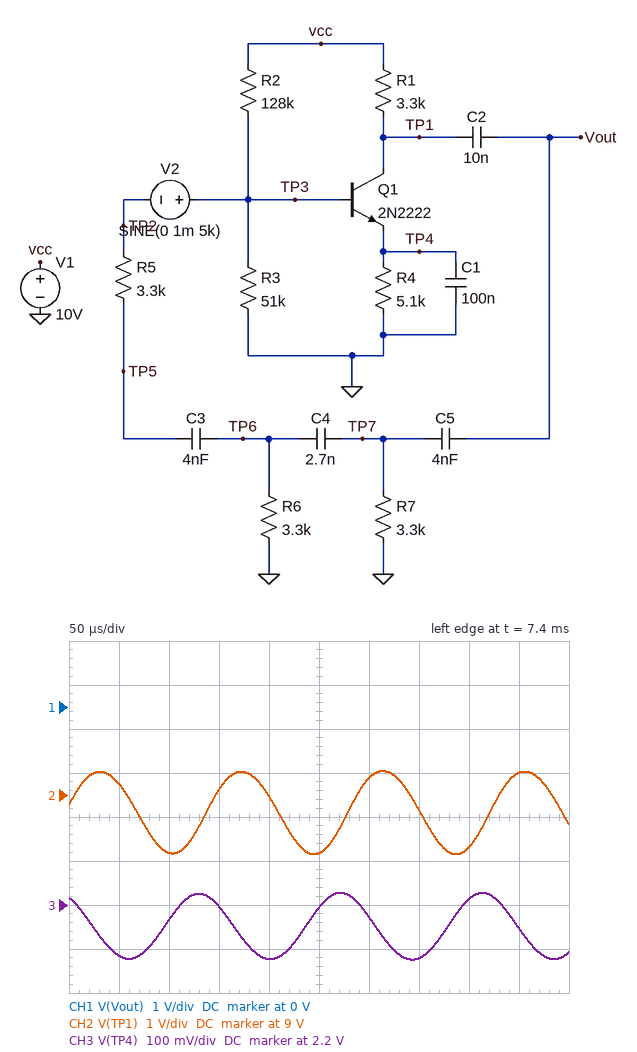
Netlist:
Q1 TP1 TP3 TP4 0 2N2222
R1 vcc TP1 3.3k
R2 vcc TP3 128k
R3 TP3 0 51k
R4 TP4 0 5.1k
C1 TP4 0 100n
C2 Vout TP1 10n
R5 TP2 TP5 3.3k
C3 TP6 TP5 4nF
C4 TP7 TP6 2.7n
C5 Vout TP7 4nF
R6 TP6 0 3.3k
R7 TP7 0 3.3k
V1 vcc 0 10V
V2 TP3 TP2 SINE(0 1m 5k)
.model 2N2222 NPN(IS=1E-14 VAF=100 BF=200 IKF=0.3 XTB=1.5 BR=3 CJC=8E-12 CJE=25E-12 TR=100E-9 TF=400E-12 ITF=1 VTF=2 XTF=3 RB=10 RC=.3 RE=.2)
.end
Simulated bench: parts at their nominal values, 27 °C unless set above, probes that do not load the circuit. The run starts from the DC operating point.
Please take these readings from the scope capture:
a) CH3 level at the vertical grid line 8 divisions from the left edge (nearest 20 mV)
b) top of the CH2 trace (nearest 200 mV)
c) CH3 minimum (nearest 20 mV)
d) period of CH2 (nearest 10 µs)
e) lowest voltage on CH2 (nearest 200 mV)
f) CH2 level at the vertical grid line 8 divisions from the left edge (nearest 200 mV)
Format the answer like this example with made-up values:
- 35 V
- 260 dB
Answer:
- 2.22 V
- 9.6 V
- 2.08 V
- 140 µs
- 7.6 V
- 7.8 V
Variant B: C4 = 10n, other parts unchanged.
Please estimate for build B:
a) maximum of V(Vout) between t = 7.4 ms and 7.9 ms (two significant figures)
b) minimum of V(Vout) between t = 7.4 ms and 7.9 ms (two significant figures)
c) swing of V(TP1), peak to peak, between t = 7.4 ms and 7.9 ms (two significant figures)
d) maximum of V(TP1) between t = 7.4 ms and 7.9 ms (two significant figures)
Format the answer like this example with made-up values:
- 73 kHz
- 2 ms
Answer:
- 6.2 V
- 6.1 V
- 100 mV
- 8.7 V
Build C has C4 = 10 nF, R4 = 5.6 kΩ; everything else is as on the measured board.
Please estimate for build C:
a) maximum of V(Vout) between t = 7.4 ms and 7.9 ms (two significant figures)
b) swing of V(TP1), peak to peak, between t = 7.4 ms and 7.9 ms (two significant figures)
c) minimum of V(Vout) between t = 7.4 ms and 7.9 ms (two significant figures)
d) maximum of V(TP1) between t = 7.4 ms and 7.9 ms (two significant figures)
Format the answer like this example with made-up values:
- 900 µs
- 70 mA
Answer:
- 6.3 V
- 96 mV
- 6.2 V
- 8.8 V
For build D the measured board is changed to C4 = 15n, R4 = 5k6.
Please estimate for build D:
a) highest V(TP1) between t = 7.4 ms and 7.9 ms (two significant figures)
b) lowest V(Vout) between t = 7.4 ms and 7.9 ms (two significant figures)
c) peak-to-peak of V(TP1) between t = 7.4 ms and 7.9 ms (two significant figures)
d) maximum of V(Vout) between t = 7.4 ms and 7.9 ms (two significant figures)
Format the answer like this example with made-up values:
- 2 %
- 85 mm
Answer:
- 8.8 V
- 6.2 V
- 63 mV
- 6.3 V
